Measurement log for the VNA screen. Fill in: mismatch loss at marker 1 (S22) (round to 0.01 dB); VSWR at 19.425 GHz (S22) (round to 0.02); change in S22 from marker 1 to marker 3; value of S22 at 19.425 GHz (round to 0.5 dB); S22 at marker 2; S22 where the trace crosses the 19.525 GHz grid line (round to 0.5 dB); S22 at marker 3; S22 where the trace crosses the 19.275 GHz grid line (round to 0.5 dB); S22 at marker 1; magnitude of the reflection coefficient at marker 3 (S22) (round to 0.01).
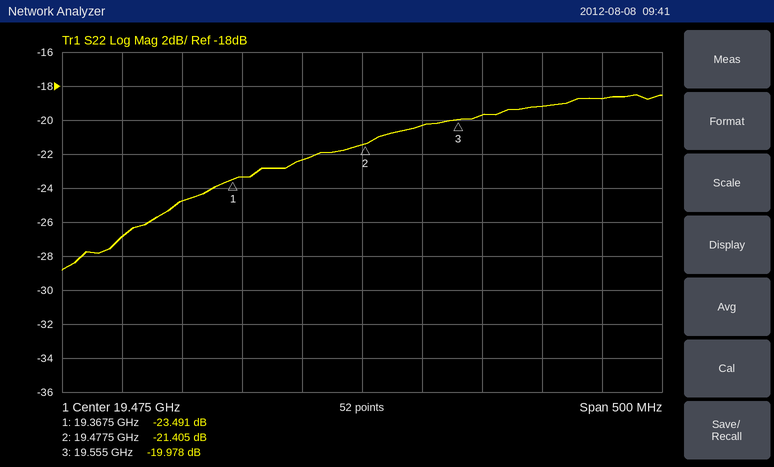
0.02 dB
1.16
3.513 dB
-22.5 dB
-21.405 dB
-20.5 dB
-19.978 dB
-27.0 dB
-23.491 dB
0.10
